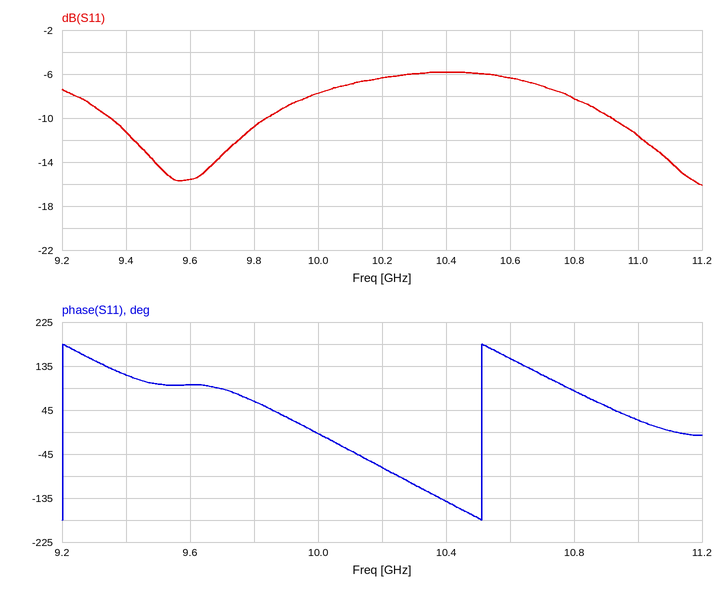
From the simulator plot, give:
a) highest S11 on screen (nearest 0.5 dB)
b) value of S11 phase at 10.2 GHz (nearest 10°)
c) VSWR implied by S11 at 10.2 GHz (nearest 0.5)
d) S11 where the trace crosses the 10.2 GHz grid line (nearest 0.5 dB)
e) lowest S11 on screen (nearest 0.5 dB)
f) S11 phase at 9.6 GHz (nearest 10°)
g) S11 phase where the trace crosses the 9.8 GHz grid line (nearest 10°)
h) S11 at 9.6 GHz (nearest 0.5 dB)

-6.0 dB
-70°
3.0
-6.5 dB
-16.0 dB
100°
60°
-15.5 dB
